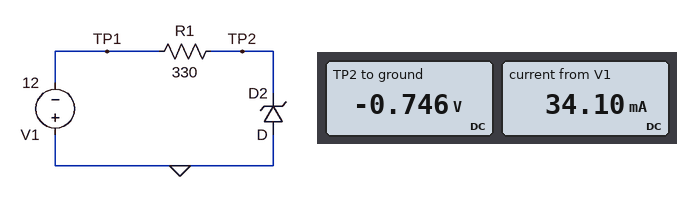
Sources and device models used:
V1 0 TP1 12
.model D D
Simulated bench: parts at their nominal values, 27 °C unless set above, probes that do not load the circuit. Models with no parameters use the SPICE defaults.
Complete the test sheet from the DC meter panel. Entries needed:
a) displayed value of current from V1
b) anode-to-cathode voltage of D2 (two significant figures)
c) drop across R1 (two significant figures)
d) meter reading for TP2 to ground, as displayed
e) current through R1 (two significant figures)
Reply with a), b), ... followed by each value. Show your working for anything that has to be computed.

a) 34.10 mA
b) 0 V - (-746 mV) = 750 mV
c) -746 mV - (-12 V) = 11 V
d) -0.746 V
e) (-746 mV - (-12 V)) / 330 Ω = 34 mA
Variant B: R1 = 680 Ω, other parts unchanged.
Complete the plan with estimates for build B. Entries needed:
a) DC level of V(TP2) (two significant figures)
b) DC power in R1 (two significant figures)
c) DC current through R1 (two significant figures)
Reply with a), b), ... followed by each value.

a) -730 mV
b) 190 mW
c) 17 mA
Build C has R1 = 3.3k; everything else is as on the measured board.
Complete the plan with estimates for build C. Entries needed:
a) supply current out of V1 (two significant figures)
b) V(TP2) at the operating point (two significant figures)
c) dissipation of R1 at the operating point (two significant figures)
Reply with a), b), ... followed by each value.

a) 3.4 mA
b) -690 mV
c) 39 mW
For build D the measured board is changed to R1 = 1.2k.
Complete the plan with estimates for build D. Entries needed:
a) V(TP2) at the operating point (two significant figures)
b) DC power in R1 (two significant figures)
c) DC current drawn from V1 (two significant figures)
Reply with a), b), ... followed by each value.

a) -710 mV
b) 110 mW
c) 9.4 mA
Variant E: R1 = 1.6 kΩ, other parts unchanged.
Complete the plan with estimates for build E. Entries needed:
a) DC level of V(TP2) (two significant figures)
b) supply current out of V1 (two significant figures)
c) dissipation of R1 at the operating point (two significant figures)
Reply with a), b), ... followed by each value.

a) -710 mV
b) 7.1 mA
c) 80 mW
